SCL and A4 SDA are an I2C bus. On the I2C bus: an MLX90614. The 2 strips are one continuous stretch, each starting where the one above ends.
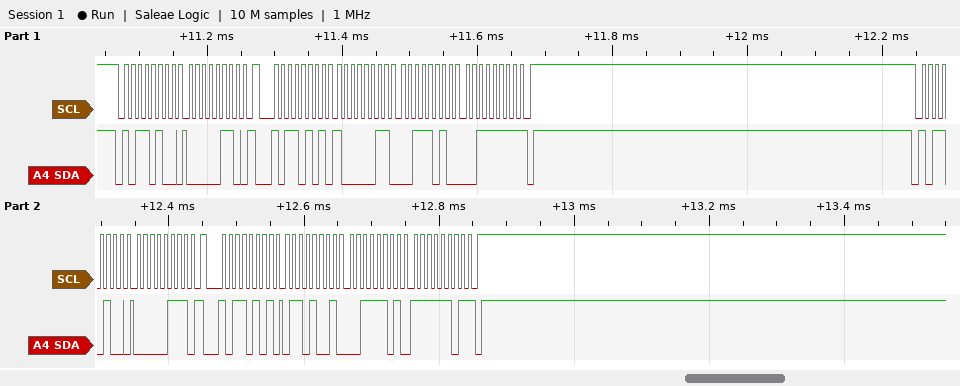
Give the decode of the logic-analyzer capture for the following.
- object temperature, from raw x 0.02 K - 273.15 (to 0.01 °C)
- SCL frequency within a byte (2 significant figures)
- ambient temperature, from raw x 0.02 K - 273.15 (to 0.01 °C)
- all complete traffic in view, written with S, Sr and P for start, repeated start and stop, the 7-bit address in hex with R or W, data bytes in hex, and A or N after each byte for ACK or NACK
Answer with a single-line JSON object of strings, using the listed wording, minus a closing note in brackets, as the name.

{"object temperature, from raw x 0.02 K - 273.15": "41.27 °C", "SCL frequency within a byte": "100 kHz", "ambient temperature, from raw x 0.02 K - 273.15": "26.43 °C", "all complete traffic in view, written with S, Sr and P for start, repeated start and stop, the 7-bit address in hex with R or W, data bytes in hex, and A or N after each byte for ACK or NACK": "S 5AW A 06 A Sr 5AR A 83 A 3A A 3F N P S 5AW A 07 A Sr 5AR A 69 A 3D A FD N P"}
